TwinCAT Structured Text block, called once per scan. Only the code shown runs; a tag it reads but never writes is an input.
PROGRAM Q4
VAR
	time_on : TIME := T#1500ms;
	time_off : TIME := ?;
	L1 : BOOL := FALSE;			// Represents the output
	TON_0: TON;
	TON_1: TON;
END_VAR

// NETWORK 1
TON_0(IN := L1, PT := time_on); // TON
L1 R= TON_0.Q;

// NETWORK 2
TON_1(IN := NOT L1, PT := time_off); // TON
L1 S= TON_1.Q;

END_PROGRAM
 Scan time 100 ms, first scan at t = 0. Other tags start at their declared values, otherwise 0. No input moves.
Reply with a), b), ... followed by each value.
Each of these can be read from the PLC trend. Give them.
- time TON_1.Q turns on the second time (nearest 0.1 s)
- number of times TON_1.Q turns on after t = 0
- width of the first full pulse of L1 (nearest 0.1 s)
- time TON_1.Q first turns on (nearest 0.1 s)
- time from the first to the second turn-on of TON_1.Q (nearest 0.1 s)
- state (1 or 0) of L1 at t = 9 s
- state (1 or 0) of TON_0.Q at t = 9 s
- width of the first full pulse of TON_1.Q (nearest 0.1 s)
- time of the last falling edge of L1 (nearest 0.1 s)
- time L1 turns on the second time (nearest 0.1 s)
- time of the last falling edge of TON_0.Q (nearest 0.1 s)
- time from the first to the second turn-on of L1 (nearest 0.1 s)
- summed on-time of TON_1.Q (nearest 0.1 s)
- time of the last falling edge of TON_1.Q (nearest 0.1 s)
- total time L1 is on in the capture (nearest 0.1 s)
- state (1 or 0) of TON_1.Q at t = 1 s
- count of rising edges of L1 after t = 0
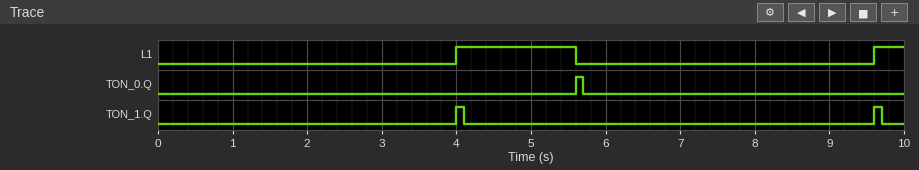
a) 9.6 s
b) 2
c) 1.6 s
d) 4.0 s
e) 5.6 s
f) 0
g) 0
h) 0.1 s
i) 5.6 s
j) 9.6 s
k) 5.7 s
l) 5.6 s
m) 0.2 s
n) 9.7 s
o) 2.0 s
p) 0
q) 2
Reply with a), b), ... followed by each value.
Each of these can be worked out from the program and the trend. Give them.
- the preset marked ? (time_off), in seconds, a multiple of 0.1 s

a) 4.0 s
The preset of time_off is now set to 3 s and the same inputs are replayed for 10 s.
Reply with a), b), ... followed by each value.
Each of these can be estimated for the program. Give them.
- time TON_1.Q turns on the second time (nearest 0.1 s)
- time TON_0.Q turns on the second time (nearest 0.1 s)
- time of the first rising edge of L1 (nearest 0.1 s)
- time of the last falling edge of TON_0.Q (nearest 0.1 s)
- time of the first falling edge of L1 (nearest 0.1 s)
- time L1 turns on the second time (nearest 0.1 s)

a) 7.6 s
b) 9.2 s
c) 3.0 s
d) 9.3 s
e) 4.6 s
f) 7.6 s
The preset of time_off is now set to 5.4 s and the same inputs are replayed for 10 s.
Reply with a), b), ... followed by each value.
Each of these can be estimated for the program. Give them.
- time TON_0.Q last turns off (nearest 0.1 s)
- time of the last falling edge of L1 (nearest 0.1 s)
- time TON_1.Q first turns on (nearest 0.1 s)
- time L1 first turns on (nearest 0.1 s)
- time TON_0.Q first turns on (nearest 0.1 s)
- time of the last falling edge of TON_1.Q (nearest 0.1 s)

a) 7.1 s
b) 7.0 s
c) 5.4 s
d) 5.4 s
e) 7.0 s
f) 5.5 s
